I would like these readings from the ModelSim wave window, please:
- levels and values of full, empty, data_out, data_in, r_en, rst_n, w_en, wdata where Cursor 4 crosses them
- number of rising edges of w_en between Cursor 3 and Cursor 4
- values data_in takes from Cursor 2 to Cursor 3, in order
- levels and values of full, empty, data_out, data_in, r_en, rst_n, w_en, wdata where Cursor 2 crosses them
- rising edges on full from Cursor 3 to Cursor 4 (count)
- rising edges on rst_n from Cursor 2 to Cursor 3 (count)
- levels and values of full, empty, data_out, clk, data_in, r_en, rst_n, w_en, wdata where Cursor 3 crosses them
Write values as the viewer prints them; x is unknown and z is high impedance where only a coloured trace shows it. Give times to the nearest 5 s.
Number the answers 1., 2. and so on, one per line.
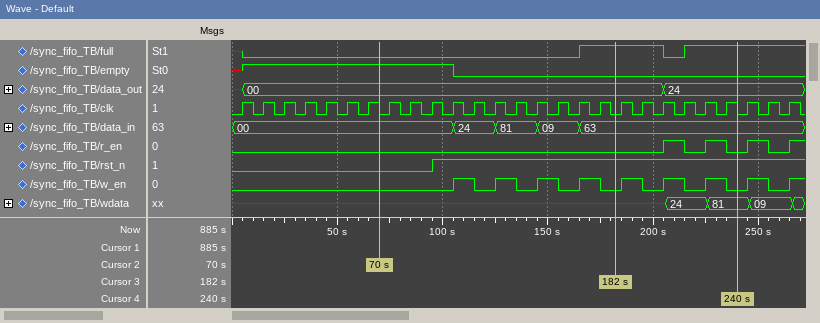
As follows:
1. full=1, empty=0, data_out=24, data_in=63, r_en=0, rst_n=1, w_en=0, wdata=81
2. 3
3. 00, 24, 81, 09, 63
4. full=0, empty=1, data_out=00, data_in=00, r_en=0, rst_n=0, w_en=0, wdata=x
5. 1
6. 1
7. full=1, empty=0, data_out=00, clk=0, data_in=63, r_en=0, rst_n=1, w_en=0, wdata=x
